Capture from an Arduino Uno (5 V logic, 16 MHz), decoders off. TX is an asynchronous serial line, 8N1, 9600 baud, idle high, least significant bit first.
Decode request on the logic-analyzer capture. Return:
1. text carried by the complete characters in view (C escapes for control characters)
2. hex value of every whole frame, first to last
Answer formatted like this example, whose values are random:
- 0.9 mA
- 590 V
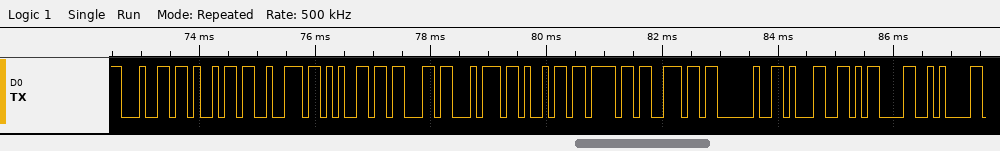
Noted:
- "direction 1\r\n"
- 0x64 0x69 0x72 0x65 0x63 0x74 0x69 0x6F 0x6E 0x20 0x31 0x0D 0x0A
